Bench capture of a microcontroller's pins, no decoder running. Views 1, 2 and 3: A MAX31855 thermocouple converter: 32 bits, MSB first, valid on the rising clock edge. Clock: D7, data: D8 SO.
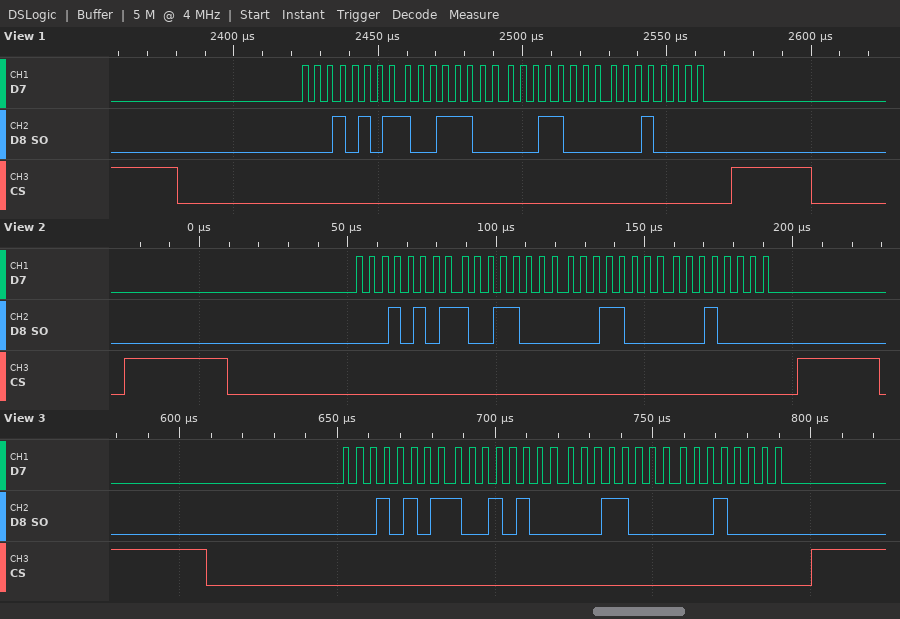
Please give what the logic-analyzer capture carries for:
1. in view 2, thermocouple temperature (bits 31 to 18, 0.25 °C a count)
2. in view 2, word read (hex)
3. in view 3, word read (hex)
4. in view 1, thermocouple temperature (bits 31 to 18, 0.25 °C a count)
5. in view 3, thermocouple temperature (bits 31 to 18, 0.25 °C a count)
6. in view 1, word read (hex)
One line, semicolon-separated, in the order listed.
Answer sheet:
345.50 °C; 0x15981810; 0x15941810; 345.75 °C; 345.25 °C; 0x159C1810
